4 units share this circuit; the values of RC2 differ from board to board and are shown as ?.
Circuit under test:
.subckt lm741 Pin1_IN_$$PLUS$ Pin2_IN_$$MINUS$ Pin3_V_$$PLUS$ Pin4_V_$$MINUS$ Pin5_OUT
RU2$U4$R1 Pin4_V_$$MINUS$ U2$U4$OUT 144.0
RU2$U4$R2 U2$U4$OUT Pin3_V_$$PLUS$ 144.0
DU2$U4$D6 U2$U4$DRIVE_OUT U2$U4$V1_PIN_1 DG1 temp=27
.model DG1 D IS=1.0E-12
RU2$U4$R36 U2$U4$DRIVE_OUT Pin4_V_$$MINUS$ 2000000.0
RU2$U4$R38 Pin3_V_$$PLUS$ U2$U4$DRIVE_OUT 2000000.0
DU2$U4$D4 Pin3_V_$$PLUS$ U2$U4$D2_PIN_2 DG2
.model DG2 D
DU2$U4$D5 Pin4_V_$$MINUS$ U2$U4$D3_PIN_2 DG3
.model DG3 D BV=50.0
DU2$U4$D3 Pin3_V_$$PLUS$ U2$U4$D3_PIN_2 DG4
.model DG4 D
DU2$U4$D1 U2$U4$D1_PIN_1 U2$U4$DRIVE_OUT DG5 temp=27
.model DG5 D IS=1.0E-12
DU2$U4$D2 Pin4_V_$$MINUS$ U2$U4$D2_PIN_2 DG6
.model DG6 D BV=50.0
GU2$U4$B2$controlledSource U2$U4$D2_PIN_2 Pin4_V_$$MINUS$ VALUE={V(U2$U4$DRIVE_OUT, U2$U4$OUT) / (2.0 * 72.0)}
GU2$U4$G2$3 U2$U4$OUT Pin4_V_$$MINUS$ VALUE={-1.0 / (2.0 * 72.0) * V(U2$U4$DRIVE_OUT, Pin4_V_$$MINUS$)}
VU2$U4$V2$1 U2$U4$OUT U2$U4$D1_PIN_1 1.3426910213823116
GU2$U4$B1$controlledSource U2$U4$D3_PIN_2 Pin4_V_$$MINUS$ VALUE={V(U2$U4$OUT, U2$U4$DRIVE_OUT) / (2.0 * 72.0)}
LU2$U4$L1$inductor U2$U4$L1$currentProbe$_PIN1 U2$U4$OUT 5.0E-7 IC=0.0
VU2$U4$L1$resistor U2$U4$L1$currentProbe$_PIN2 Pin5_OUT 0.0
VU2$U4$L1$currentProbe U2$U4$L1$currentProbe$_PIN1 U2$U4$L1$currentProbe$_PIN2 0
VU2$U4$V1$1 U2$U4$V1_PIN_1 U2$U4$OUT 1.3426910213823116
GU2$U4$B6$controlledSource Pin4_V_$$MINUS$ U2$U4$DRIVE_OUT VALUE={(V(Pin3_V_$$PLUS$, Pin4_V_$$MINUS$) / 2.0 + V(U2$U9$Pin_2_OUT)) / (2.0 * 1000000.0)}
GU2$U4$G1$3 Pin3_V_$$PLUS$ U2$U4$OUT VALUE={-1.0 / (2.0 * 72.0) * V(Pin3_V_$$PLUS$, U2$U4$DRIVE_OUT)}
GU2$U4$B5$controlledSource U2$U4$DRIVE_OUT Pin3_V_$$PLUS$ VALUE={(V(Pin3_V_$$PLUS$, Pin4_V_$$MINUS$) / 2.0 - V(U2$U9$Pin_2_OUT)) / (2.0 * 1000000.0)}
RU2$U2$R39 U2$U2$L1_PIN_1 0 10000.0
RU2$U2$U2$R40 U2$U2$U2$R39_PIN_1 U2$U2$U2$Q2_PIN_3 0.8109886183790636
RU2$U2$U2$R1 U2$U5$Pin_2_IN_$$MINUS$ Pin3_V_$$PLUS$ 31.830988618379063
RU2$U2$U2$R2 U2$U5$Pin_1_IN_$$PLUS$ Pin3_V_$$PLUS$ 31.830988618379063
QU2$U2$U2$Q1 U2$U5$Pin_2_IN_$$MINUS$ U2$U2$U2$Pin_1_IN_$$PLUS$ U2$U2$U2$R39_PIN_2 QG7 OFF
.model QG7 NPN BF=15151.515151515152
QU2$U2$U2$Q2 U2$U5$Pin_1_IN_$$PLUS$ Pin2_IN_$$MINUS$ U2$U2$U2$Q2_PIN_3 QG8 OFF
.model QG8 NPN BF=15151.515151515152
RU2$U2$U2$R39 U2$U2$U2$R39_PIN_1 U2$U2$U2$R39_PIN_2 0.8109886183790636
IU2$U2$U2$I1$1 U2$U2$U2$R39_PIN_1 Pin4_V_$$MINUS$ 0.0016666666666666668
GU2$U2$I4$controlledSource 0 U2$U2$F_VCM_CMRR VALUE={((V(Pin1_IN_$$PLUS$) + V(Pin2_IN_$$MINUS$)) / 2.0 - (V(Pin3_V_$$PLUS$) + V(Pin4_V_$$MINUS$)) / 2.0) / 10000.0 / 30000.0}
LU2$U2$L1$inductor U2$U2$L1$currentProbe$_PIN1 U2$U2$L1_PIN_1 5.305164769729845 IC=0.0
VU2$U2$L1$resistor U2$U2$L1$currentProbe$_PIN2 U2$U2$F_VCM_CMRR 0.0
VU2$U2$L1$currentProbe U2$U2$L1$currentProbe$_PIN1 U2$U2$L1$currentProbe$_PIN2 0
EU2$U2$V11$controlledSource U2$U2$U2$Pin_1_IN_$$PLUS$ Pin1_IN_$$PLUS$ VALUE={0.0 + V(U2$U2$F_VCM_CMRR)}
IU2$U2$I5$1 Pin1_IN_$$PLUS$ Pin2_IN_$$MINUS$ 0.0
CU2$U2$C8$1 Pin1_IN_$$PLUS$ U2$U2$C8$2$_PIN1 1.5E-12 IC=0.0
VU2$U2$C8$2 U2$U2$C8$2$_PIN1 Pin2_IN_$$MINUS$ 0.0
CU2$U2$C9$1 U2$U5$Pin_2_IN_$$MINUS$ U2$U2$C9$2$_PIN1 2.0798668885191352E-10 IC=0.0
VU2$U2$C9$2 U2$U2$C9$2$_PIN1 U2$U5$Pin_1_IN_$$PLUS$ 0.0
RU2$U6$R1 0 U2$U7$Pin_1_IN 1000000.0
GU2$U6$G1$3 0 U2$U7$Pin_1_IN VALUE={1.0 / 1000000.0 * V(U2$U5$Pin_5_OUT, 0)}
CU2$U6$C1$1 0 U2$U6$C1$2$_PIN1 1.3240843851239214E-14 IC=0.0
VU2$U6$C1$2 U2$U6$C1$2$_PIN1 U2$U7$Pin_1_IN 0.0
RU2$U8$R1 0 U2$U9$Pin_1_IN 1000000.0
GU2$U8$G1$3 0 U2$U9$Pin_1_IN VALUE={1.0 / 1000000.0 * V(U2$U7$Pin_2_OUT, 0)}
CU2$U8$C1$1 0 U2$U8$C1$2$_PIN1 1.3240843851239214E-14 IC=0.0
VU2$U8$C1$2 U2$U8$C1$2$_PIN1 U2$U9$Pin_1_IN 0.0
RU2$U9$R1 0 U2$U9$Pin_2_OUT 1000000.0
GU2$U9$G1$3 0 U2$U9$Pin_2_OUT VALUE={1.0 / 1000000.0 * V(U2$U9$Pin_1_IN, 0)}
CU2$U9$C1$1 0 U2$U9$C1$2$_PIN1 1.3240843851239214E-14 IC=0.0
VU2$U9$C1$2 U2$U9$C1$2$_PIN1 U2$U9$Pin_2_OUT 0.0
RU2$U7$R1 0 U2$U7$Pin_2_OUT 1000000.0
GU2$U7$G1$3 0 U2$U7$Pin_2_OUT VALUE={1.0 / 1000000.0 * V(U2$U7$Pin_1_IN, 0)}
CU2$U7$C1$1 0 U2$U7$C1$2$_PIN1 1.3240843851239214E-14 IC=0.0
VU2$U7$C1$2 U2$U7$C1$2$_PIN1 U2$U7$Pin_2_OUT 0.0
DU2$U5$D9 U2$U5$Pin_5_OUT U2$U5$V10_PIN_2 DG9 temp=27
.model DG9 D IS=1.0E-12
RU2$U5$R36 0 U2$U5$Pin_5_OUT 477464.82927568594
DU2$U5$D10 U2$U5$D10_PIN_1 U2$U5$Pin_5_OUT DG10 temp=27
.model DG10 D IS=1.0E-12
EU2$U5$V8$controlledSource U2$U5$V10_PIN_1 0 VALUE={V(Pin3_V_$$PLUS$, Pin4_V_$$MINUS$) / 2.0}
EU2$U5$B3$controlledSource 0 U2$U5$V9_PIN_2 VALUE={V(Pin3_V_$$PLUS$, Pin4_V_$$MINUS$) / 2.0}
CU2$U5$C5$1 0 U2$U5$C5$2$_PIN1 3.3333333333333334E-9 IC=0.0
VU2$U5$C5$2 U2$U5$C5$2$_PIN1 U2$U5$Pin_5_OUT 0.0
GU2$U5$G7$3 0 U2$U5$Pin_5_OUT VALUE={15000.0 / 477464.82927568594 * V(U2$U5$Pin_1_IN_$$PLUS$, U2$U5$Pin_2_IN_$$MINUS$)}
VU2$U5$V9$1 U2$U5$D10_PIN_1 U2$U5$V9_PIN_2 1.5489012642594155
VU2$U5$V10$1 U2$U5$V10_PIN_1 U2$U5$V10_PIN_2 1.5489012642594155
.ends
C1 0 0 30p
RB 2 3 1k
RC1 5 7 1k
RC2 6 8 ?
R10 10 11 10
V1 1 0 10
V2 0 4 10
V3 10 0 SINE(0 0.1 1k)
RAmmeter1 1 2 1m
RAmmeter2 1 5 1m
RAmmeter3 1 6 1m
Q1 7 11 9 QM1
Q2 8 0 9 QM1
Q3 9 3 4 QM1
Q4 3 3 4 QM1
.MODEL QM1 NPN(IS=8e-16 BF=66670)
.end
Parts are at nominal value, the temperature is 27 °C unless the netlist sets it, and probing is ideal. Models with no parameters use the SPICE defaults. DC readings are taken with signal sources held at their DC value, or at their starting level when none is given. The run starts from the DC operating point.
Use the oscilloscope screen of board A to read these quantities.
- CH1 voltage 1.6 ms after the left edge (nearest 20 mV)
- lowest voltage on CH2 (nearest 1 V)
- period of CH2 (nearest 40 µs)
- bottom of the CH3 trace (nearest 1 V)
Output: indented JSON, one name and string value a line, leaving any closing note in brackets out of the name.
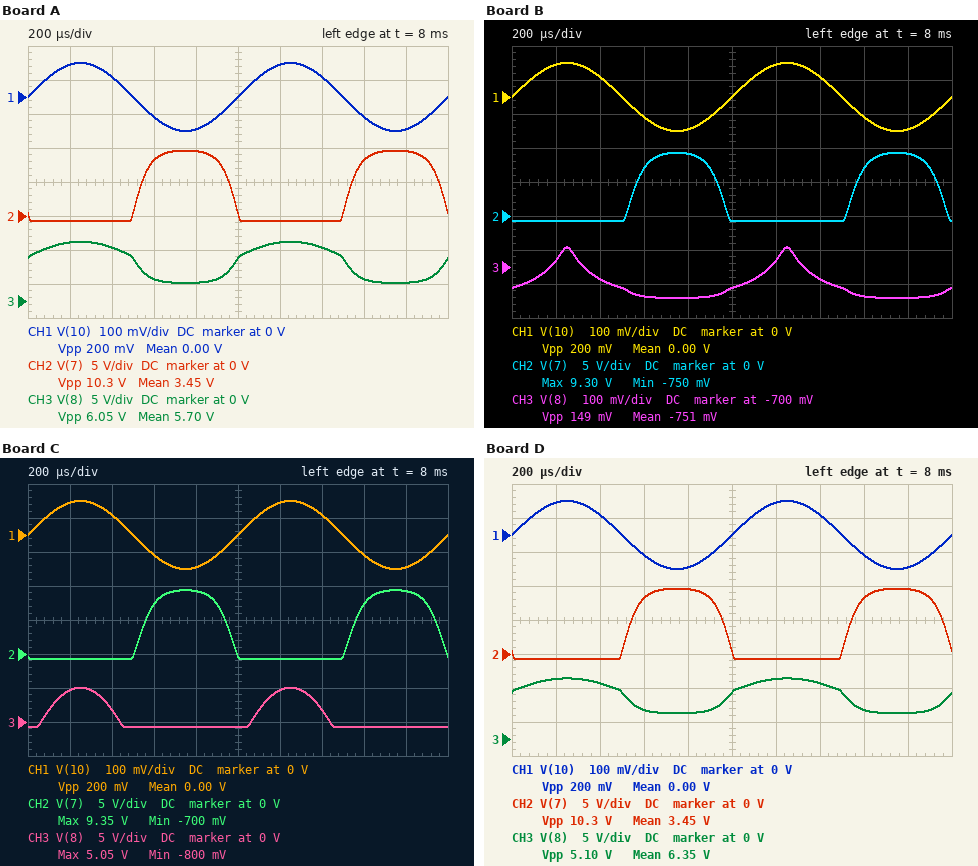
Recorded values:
{
  "CH1 voltage 1.6 ms after the left edge": "-60 mV",
  "lowest voltage on CH2": "-1 V",
  "period of CH2": "1.00 ms",
  "bottom of the CH3 trace": "3 V"
}
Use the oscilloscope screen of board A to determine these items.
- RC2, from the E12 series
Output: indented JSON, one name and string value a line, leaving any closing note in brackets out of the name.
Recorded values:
{
  "RC2, from the E12 series": "390 Ω"
}
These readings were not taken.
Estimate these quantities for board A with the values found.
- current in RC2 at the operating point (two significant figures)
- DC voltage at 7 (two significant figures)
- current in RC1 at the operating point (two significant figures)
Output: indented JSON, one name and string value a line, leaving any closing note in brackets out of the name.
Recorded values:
{
  "current in RC2 at the operating point": "9.6 mA",
  "DC voltage at 7": "400 mV",
  "current in RC1 at the operating point": "9.6 mA"
}
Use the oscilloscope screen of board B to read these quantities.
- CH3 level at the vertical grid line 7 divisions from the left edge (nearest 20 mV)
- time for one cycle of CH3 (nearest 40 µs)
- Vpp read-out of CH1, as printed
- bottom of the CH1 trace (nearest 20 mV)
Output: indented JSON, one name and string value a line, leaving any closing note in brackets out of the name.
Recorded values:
{
  "CH3 level at the vertical grid line 7 divisions from the left edge": "-740 mV",
  "time for one cycle of CH3": "1.00 ms",
  "Vpp read-out of CH1, as printed": "200 mV",
  "bottom of the CH1 trace": "-100 mV"
}
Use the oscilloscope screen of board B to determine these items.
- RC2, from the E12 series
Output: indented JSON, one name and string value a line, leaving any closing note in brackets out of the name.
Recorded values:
{
  "RC2, from the E12 series": "3.3 kΩ"
}
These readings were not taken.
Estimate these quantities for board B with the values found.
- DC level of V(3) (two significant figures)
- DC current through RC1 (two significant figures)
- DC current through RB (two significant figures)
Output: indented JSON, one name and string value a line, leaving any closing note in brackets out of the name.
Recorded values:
{
  "DC level of V(3)": "-9.2 V",
  "DC current through RC1": "11 mA",
  "DC current through RB": "19 mA"
}
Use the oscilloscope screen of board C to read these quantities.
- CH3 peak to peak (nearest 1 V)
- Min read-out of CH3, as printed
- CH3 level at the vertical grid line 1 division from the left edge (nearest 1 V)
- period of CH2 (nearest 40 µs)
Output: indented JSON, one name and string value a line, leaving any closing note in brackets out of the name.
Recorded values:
{
  "CH3 peak to peak": "6 V",
  "Min read-out of CH3, as printed": "-800 mV",
  "CH3 level at the vertical grid line 1 division from the left edge": "5 V",
  "period of CH2": "1.00 ms"
}
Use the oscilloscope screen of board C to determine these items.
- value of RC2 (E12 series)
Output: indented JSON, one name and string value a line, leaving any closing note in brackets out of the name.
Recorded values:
{
  "value of RC2": "1.5 kΩ"
}
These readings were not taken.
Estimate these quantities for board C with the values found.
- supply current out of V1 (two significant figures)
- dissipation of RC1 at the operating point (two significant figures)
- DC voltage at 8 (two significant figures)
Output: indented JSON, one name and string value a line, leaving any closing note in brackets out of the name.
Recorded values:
{
  "supply current out of V1": "37 mA",
  "dissipation of RC1 at the operating point": "110 mW",
  "DC voltage at 8": "-730 mV"
}
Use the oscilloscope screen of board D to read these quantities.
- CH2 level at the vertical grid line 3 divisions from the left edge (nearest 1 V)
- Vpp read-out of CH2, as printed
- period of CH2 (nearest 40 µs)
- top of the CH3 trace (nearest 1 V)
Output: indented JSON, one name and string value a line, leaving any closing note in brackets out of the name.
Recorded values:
{
  "CH2 level at the vertical grid line 3 divisions from the left edge": "8 V",
  "Vpp read-out of CH2, as printed": "10.3 V",
  "period of CH2": "1.00 ms",
  "top of the CH3 trace": "9 V"
}
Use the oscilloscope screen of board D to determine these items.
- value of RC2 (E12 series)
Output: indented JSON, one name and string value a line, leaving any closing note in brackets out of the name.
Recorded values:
{
  "value of RC2": "330 Ω"
}
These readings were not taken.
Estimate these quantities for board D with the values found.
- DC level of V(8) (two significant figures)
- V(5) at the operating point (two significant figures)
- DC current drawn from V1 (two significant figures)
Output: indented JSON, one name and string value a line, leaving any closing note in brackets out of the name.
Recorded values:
{
  "DC level of V(8)": "6.8 V",
  "V(5) at the operating point": "10 V",
  "DC current drawn from V1": "38 mA"
}
